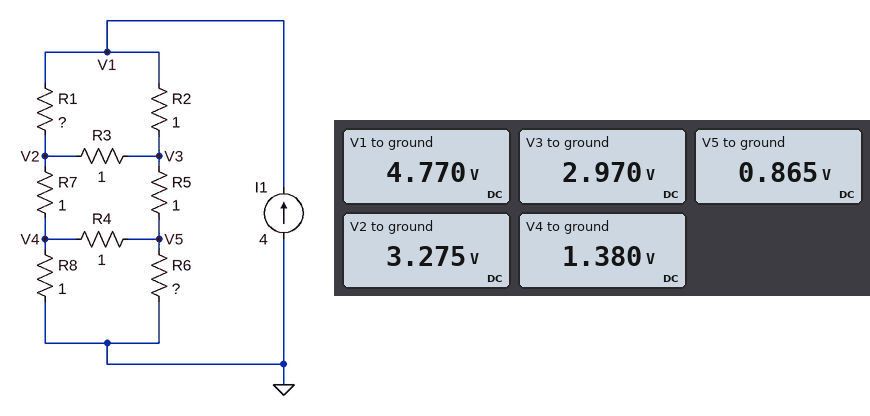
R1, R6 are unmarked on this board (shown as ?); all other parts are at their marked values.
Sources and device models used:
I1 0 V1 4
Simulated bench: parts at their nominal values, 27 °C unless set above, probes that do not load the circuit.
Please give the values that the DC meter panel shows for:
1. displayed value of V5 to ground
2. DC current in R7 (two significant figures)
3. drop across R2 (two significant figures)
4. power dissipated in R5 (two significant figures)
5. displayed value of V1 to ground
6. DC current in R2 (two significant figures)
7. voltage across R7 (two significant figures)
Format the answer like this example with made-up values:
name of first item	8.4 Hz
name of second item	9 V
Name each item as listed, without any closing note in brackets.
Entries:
displayed value of V5 to ground	0.865 V
DC current in R7	1.9 A
drop across R2	1.8 V
power dissipated in R5	4.4 W
displayed value of V1 to ground	4.770 V
DC current in R2	1.8 A
voltage across R7	1.9 V
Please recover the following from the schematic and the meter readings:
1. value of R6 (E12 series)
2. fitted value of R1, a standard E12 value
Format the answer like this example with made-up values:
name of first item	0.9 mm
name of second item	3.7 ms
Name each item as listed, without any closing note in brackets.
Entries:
value of R6	0.33 Ω
fitted value of R1, a standard E12 value	0.68 Ω
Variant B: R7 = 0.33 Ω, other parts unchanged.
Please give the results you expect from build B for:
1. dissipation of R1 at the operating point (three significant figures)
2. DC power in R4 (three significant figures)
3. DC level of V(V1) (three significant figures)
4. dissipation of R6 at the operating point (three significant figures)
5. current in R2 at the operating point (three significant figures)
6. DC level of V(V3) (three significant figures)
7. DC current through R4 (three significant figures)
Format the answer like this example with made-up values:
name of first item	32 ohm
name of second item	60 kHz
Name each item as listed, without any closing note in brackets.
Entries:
dissipation of R1 at the operating point	3.87 W
DC power in R4	643 mW
DC level of V(V1)	4.01 V
dissipation of R6 at the operating point	1.91 W
current in R2 at the operating point	1.61 A
DC level of V(V3)	2.40 V
DC current through R4	802 mA
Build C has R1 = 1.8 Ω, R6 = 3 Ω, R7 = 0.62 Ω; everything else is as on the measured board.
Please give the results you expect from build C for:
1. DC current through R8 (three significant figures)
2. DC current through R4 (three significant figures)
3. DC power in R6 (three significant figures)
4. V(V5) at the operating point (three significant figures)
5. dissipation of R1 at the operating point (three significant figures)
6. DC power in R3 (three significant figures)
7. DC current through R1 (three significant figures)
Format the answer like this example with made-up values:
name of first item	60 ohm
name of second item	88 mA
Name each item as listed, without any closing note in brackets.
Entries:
DC current through R8	2.87 A
DC current through R4	511 mA
DC power in R6	3.82 W
V(V5) at the operating point	3.38 V
dissipation of R1 at the operating point	5.04 W
DC power in R3	472 mW
DC current through R1	1.67 A
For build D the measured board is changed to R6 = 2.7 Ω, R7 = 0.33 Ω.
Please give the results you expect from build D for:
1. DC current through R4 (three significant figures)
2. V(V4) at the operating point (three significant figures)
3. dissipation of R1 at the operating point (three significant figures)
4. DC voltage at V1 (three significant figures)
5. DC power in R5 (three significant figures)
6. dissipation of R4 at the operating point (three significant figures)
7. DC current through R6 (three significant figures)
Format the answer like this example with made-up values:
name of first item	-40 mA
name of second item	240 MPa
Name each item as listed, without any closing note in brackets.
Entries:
DC current through R4	62.9 mA
V(V4) at the operating point	2.90 V
dissipation of R1 at the operating point	4.43 W
DC voltage at V1	5.57 V
DC power in R5	1.35 W
dissipation of R4 at the operating point	3.96 mW
DC current through R6	1.10 A
